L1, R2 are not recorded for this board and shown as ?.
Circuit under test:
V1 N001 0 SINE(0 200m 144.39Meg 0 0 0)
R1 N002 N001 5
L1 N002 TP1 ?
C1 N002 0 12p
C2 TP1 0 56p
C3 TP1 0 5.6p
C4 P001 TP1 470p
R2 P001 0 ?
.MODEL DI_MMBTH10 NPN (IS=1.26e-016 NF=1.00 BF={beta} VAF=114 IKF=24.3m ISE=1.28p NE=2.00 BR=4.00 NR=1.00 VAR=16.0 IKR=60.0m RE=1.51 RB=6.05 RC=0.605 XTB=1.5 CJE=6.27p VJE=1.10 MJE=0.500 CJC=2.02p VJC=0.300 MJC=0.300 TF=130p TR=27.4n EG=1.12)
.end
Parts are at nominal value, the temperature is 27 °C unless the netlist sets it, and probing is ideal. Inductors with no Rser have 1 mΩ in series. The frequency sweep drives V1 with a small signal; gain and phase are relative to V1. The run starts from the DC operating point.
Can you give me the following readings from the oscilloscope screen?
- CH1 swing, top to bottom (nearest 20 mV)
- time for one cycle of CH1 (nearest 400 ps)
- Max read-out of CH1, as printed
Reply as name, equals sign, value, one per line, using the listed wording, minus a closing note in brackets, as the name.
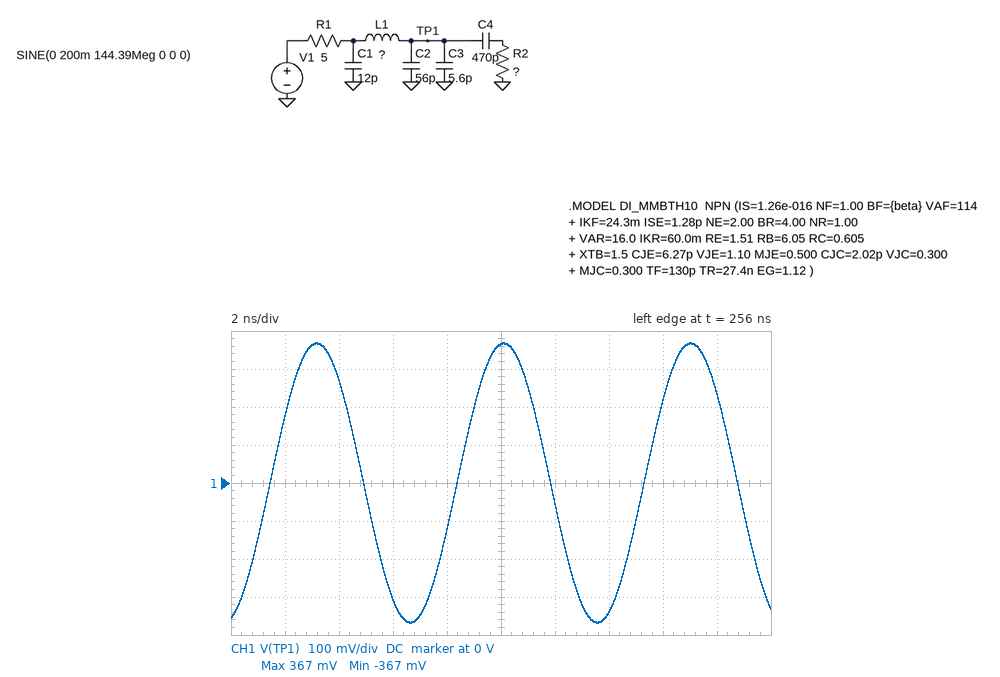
CH1 swing, top to bottom = 740 mV
time for one cycle of CH1 = 6.8 ns
Max read-out of CH1, as printed = 367 mV
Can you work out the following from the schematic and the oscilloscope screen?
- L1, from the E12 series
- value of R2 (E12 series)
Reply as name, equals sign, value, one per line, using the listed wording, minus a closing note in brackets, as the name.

L1, from the E12 series = 18 nH
value of R2 = 68 Ω
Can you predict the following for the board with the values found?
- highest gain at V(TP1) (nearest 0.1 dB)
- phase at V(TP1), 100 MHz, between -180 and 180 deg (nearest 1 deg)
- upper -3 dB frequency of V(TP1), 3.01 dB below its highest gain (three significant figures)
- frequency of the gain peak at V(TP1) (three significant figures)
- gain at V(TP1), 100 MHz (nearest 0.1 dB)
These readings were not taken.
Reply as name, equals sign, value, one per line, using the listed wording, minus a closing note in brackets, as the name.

highest gain at V(TP1) = 5.3 dB
phase at V(TP1), 100 MHz, between -180 and 180 deg = -32 deg
upper -3 dB frequency of V(TP1), 3.01 dB below its highest gain = 184 MHz
frequency of the gain peak at V(TP1) = 146 MHz
gain at V(TP1), 100 MHz = 2.7 dB
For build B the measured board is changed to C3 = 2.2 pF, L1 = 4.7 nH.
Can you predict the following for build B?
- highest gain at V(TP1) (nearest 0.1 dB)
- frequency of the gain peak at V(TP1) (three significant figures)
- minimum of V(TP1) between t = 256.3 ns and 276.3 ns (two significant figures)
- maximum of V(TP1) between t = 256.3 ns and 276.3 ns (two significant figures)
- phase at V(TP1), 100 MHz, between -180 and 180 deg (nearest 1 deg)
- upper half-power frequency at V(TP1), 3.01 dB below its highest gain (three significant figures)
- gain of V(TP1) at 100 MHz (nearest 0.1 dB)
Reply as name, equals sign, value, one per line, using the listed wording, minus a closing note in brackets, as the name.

highest gain at V(TP1) = 3.3 dB
frequency of the gain peak at V(TP1) = 286 MHz
minimum of V(TP1) between t = 256.3 ns and 276.3 ns = -220 mV
maximum of V(TP1) between t = 256.3 ns and 276.3 ns = 220 mV
phase at V(TP1), 100 MHz, between -180 and 180 deg = -15 deg
upper half-power frequency at V(TP1), 3.01 dB below its highest gain = 386 MHz
gain of V(TP1) at 100 MHz = 0 dB
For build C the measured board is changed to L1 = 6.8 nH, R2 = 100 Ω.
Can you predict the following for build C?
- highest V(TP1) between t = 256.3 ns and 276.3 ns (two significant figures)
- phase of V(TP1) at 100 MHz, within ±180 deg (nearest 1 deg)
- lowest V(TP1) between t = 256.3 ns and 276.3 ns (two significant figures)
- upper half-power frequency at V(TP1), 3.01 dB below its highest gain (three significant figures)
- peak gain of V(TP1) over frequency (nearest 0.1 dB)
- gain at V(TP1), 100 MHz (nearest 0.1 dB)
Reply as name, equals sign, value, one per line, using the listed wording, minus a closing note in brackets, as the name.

highest V(TP1) between t = 256.3 ns and 276.3 ns = 250 mV
phase of V(TP1) at 100 MHz, within ±180 deg = -17 deg
lowest V(TP1) between t = 256.3 ns and 276.3 ns = -250 mV
upper half-power frequency at V(TP1), 3.01 dB below its highest gain = 303 MHz
peak gain of V(TP1) over frequency = 4.8 dB
gain at V(TP1), 100 MHz = 0.7 dB
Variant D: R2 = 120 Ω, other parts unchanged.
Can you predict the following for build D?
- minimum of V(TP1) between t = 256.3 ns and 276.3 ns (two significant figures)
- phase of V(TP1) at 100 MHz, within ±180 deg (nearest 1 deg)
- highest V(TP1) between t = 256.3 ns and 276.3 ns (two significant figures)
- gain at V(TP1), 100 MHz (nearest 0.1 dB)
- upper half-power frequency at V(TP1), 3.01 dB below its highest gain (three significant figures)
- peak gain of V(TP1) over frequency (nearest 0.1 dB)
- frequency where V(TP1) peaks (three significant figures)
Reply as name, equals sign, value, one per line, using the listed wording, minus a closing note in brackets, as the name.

minimum of V(TP1) between t = 256.3 ns and 276.3 ns = -460 mV
phase of V(TP1) at 100 MHz, within ±180 deg = -27 deg
highest V(TP1) between t = 256.3 ns and 276.3 ns = 460 mV
gain at V(TP1), 100 MHz = 3.4 dB
upper half-power frequency at V(TP1), 3.01 dB below its highest gain = 179 MHz
peak gain of V(TP1) over frequency = 7.2 dB
frequency where V(TP1) peaks = 148 MHz
